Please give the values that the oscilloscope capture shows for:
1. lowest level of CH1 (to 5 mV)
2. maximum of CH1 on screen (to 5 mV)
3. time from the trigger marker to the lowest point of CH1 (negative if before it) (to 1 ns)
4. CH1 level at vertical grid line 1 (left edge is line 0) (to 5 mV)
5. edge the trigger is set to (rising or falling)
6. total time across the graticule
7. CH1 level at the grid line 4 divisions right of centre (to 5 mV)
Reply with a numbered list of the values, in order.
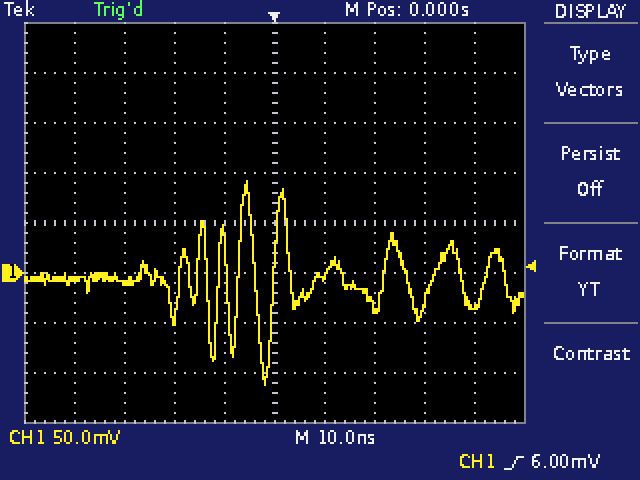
1. -110 mV
2. 90 mV
3. -2 ns
4. -5 mV
5. rising
6. 100 ns
7. -35 mV
